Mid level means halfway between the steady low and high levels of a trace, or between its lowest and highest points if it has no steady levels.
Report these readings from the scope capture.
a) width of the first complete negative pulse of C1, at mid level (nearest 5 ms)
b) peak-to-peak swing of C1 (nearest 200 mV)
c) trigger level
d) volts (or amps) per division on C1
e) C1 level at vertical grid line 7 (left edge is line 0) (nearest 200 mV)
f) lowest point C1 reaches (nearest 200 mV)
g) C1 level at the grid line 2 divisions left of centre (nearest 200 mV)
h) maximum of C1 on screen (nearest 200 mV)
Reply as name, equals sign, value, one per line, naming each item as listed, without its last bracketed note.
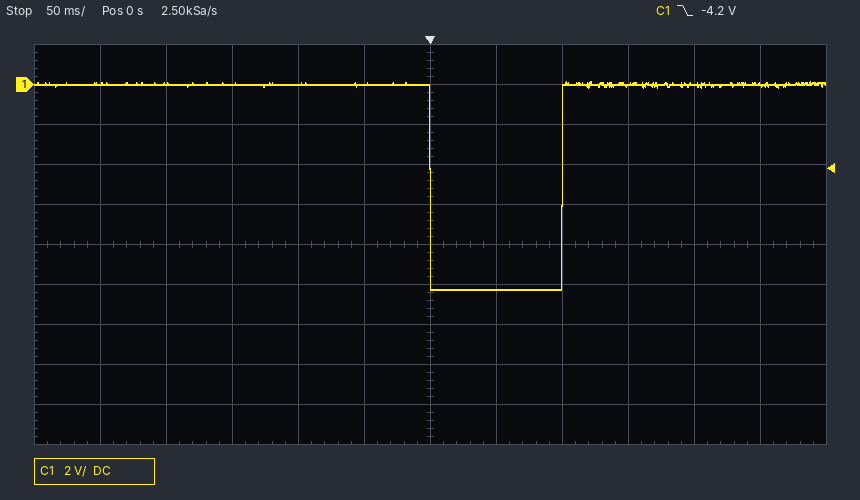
width of the first complete negative pulse of C1, at mid level = 100 ms
peak-to-peak swing of C1 = 10.4 V
trigger level = -4.2 V
volts (or amps) per division on C1 = 2 V
C1 level at vertical grid line 7 (left edge is line 0) = -10.2 V
lowest point C1 reaches = -10.2 V
C1 level at the grid line 2 divisions left of centre = 0.0 V
maximum of C1 on screen = 200 mV
